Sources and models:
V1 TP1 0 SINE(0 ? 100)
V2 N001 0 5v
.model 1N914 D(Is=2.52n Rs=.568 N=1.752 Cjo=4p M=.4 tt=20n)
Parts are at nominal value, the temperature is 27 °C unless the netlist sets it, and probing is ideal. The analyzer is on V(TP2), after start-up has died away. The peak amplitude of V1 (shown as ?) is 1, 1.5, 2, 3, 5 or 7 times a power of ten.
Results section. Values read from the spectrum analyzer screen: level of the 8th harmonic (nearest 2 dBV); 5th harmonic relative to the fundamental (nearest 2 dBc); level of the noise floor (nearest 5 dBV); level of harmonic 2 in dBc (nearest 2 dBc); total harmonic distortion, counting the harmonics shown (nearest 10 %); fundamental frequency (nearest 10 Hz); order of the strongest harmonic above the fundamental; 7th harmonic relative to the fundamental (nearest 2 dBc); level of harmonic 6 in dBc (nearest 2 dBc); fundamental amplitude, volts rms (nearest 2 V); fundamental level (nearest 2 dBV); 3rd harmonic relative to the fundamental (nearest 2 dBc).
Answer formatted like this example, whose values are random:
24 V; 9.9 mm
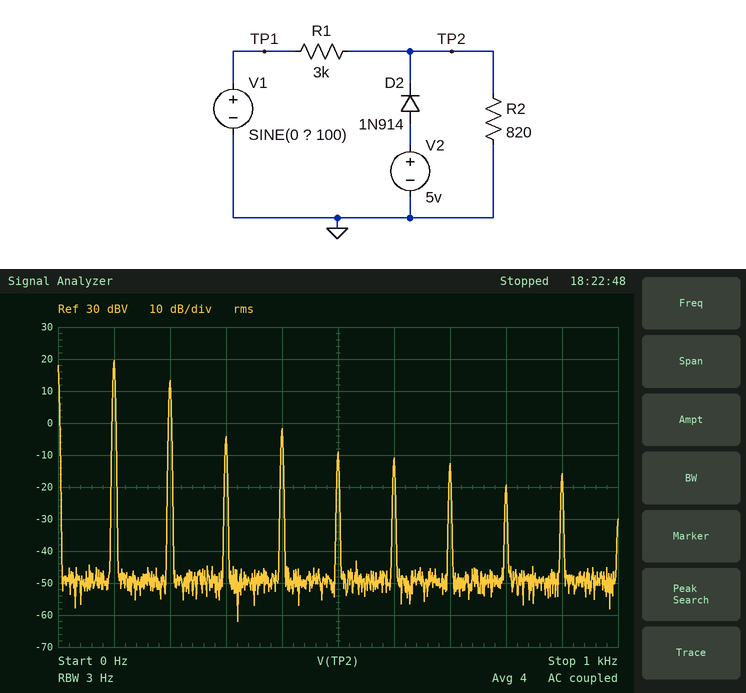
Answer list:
-20 dBV; -28 dBc; -50 dBV; -6 dBc; 50 %; 100 Hz; 2; -32 dBc; -30 dBc; 10 V; 20 dBV; -24 dBc
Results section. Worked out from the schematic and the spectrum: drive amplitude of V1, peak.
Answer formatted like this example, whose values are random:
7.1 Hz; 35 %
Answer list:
150 V
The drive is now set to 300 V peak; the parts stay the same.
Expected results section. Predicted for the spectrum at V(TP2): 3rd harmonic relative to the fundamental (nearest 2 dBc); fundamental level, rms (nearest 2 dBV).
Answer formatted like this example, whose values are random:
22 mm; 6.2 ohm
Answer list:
-30 dBc; 26 dBV
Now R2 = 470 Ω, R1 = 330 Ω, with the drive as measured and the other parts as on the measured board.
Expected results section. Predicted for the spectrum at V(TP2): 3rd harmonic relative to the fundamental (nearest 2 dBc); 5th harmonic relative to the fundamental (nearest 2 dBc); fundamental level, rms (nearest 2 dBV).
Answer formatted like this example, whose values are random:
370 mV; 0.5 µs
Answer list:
-34 dBc; -38 dBc; 30 dBV
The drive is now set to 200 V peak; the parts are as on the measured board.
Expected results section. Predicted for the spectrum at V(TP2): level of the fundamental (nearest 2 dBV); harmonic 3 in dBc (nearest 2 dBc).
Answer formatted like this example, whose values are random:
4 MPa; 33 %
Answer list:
22 dBV; -26 dBc
